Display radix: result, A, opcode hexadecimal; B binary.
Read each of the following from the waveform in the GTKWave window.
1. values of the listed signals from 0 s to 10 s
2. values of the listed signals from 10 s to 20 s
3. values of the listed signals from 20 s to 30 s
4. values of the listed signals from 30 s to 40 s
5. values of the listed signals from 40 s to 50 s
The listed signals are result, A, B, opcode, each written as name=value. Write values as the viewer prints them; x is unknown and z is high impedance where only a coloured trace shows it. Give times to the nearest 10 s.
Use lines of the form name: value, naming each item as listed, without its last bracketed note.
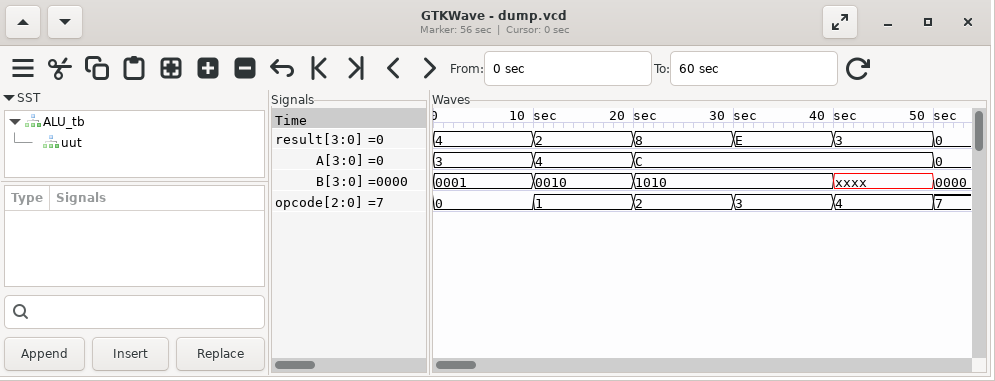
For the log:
values of the listed signals from 0 s to 10 s: result=4, A=3, B=0001, opcode=0
values of the listed signals from 10 s to 20 s: result=2, A=4, B=0010, opcode=1
values of the listed signals from 20 s to 30 s: result=8, A=C, B=1010, opcode=2
values of the listed signals from 30 s to 40 s: result=E, A=C, B=1010, opcode=3
values of the listed signals from 40 s to 50 s: result=3, A=C, B=xxxx, opcode=4
